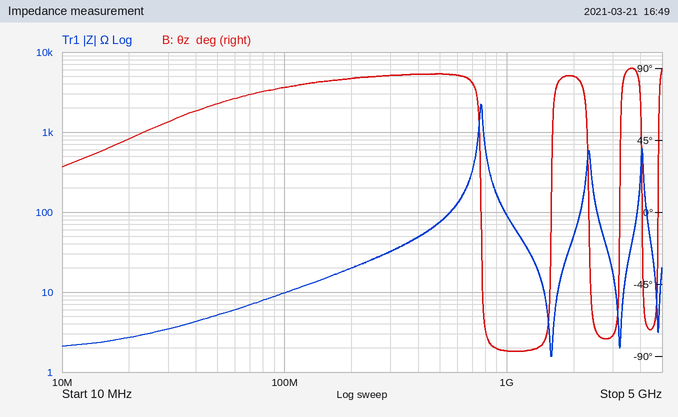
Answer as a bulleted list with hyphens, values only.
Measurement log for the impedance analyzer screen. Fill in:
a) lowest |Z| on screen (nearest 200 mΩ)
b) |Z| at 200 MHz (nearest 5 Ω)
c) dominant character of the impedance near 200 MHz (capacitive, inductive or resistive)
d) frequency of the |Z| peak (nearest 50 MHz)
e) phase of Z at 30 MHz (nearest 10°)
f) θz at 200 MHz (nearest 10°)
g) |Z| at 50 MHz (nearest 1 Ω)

- 1.6 Ω
- 20 Ω
- inductive
- 750 MHz
- 60°
- 80°
- 5 Ω
